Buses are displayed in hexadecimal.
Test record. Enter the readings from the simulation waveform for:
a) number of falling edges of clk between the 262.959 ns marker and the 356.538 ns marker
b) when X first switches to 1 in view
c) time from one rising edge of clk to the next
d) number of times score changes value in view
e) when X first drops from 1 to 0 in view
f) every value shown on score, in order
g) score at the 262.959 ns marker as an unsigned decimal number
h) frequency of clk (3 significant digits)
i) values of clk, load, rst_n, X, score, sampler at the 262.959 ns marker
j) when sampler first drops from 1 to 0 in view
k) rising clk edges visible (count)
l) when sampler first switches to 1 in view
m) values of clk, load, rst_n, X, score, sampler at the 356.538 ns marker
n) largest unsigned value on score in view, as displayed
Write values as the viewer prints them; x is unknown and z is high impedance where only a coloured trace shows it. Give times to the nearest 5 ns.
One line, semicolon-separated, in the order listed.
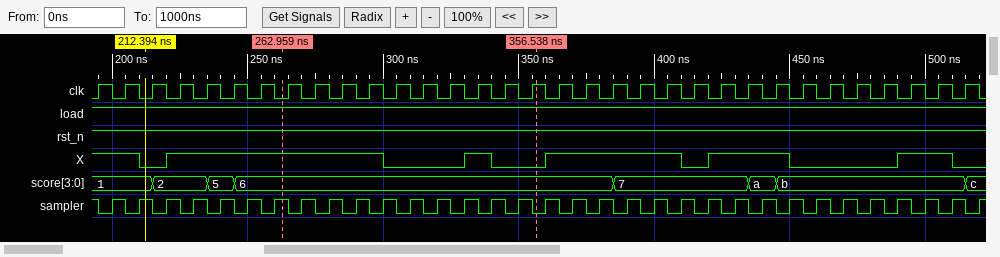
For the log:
9; 220 ns; 10 ns; 7; 210 ns; 1, 2, 5, 6, 7, a, b, c; 6; 100 MHz; clk=0, load=1, rst_n=1, X=1, score=6, sampler=1; 195 ns; 33; 200 ns; clk=1, load=1, rst_n=1, X=0, score=6, sampler=0; c
